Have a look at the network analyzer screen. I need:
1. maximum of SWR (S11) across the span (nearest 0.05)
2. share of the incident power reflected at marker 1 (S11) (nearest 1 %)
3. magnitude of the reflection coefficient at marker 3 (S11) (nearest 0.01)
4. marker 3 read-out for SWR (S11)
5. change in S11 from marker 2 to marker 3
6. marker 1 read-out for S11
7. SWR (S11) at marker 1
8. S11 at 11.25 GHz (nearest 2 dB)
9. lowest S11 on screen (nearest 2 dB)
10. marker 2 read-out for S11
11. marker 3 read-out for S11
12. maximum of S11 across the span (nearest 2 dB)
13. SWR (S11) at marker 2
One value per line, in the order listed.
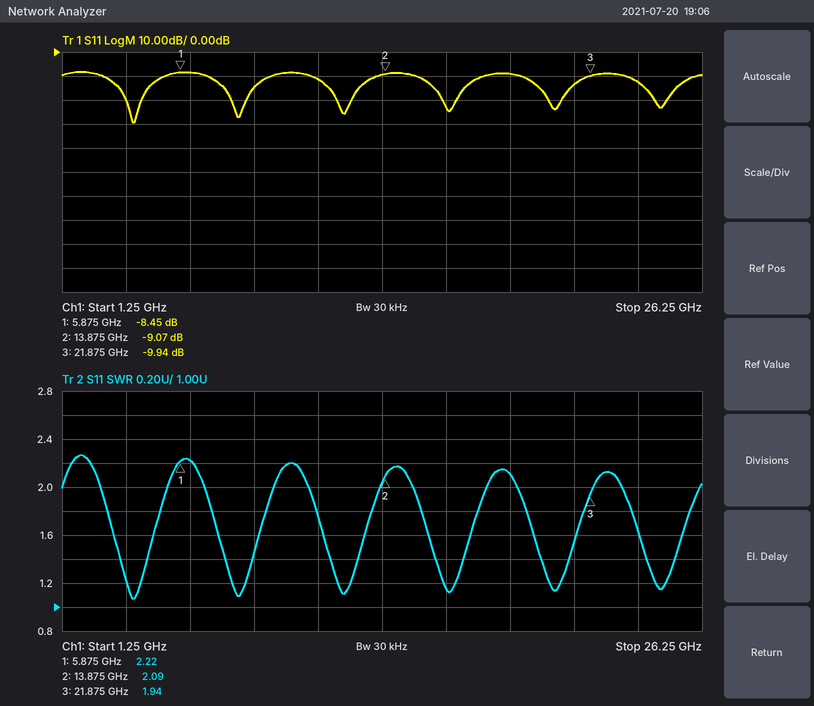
2.25
14 %
0.32
1.94
-0.87 dB
-8.45 dB
2.22
-12 dB
-30 dB
-9.07 dB
-9.94 dB
-8 dB
2.09
